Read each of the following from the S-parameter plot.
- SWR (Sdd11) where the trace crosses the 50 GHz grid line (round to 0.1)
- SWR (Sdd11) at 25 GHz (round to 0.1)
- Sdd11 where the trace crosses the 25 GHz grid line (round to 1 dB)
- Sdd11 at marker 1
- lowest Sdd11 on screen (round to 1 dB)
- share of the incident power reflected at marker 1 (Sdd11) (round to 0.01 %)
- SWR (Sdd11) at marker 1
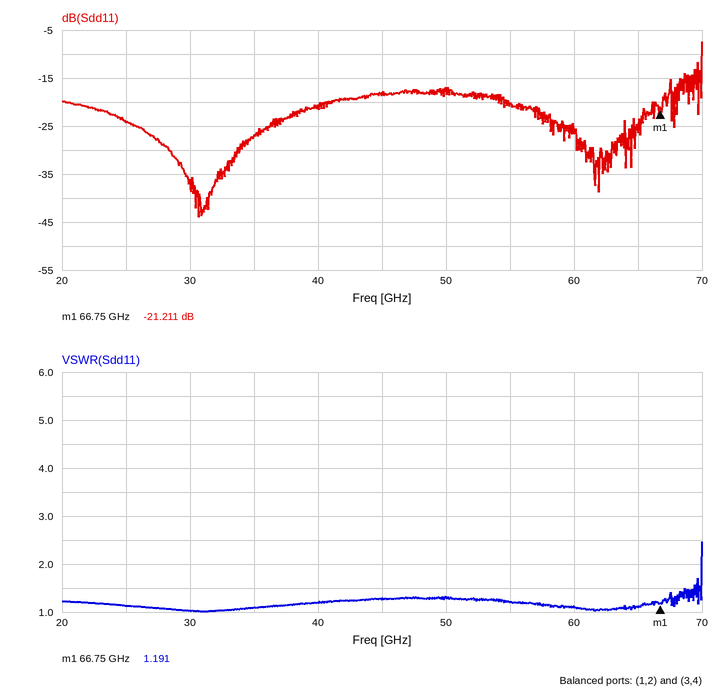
1.3
1.1
-24 dB
-21.211 dB
-44 dB
0.76 %
1.191
